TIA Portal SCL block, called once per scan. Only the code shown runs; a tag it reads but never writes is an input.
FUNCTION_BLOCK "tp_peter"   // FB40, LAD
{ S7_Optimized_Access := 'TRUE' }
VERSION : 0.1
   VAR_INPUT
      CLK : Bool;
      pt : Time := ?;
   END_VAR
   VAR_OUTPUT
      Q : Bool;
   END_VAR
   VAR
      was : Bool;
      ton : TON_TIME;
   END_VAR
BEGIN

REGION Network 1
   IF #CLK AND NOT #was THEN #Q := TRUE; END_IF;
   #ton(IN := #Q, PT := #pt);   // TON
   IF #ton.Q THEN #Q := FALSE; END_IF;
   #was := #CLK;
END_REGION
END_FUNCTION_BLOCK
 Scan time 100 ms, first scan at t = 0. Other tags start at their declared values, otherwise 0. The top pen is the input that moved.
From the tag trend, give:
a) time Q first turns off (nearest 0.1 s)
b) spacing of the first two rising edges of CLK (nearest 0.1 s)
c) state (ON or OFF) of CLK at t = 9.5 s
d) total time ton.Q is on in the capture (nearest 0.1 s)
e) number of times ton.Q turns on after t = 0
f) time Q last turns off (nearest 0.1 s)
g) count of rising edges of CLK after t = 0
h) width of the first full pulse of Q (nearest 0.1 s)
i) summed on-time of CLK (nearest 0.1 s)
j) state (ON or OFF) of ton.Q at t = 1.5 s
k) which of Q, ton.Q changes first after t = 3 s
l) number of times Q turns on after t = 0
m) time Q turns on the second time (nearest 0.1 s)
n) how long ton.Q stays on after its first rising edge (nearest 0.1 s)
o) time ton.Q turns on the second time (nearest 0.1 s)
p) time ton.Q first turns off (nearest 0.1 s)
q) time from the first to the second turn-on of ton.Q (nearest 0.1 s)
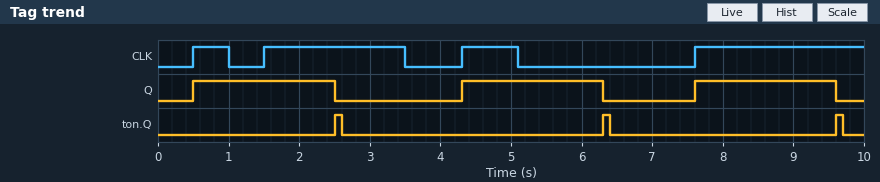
2.5 s
1.0 s
ON
0.3 s
3
9.6 s
4
2.0 s
5.7 s
OFF
Q
3
4.3 s
0.1 s
6.3 s
2.6 s
3.8 s
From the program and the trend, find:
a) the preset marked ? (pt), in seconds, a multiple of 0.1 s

2.0 s
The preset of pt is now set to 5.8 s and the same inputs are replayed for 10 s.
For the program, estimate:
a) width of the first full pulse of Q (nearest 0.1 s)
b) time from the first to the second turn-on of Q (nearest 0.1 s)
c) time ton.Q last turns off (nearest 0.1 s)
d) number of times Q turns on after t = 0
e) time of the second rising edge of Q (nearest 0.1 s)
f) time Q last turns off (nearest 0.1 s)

5.8 s
7.1 s
6.4 s
2
7.6 s
6.3 s
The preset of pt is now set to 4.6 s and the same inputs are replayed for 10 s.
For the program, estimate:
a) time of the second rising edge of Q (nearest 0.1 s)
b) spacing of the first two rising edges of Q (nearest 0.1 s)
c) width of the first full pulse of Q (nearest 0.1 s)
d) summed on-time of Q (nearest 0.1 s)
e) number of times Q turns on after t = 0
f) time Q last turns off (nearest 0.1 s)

7.6 s
7.1 s
4.6 s
7.0 s
2
5.1 s
